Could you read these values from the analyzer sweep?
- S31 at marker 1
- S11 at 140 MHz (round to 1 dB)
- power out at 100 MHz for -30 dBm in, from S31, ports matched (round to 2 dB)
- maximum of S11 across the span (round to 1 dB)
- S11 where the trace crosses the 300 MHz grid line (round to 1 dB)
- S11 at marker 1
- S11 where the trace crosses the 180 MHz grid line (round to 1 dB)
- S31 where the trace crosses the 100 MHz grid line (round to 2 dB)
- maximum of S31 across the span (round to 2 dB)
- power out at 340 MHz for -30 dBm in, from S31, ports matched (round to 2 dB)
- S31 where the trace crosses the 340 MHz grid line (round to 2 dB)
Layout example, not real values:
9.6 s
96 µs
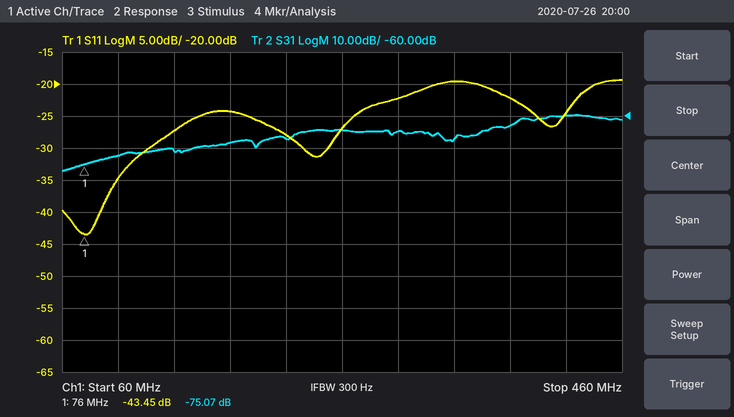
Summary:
-75.07 dB
-27 dB
-102 dBm
-19 dB
-22 dB
-43.45 dB
-24 dB
-72 dB
-60 dB
-98 dBm
-68 dB
